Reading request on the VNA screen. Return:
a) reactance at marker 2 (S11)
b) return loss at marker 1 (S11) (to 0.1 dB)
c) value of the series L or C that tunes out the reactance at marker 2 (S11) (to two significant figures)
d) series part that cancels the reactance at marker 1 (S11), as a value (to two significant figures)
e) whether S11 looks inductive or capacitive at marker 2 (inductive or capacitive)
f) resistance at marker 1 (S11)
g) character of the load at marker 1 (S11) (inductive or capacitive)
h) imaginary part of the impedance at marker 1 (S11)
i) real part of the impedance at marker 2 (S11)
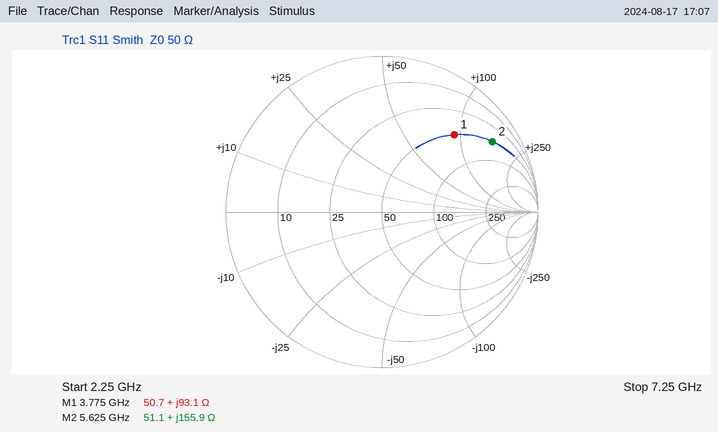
+155.9 Ω
3.4 dB
180 fF
450 fF
inductive
50.7 Ω
inductive
+93.1 Ω
51.1 Ω
